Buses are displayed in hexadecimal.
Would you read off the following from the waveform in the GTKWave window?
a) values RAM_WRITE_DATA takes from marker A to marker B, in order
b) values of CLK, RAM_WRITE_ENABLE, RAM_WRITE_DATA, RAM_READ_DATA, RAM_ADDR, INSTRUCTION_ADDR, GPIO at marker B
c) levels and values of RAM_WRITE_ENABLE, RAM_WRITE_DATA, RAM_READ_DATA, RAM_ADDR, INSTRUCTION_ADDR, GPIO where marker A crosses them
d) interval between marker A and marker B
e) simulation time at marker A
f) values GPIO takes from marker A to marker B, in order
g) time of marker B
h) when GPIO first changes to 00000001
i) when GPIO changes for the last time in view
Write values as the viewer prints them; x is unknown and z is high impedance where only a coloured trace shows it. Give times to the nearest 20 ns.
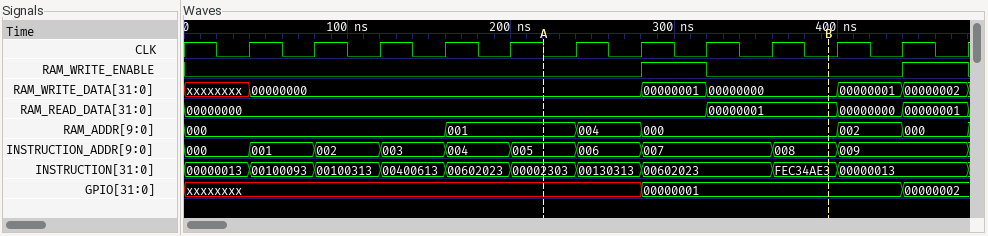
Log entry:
00000000, 00000001, 00000000
CLK=0, RAM_WRITE_ENABLE=0, RAM_WRITE_DATA=00000000, RAM_READ_DATA=00000001, RAM_ADDR=000, INSTRUCTION_ADDR=008, GPIO=00000001
RAM_WRITE_ENABLE=0, RAM_WRITE_DATA=00000000, RAM_READ_DATA=00000000, RAM_ADDR=001, INSTRUCTION_ADDR=005, GPIO=xxxxxxxx
180 ns
220 ns
xxxxxxxx, 00000001
400 ns
280 ns
440 ns
